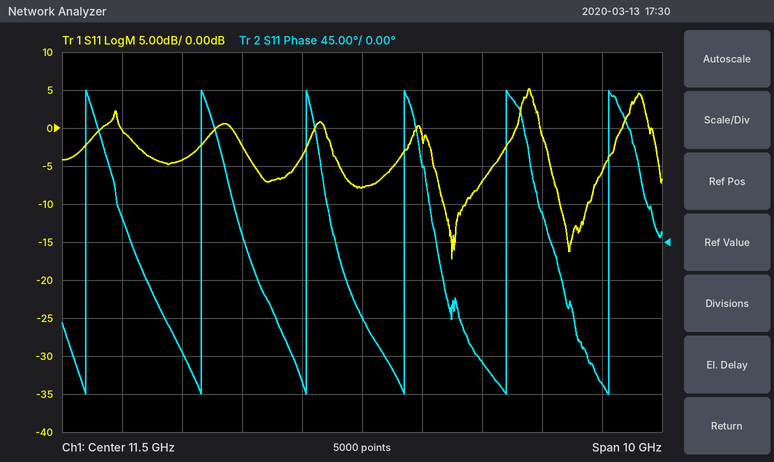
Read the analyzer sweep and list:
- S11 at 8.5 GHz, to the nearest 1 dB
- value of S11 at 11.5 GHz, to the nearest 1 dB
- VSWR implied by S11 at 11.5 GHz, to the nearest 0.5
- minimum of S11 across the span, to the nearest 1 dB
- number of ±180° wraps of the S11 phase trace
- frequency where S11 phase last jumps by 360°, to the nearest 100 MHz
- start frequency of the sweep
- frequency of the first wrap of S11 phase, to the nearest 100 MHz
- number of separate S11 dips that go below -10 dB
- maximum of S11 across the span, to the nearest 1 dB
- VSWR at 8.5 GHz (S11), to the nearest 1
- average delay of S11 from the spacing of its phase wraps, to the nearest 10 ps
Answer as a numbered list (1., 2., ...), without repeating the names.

1. -4 dB
2. -8 dB
3. 2.5
4. -17 dB
5. 6
6. 15.6 GHz
7. 6.5 GHz
8. 6.9 GHz
9. 2
10. 5 dB
11. 4
12. 570 ps
